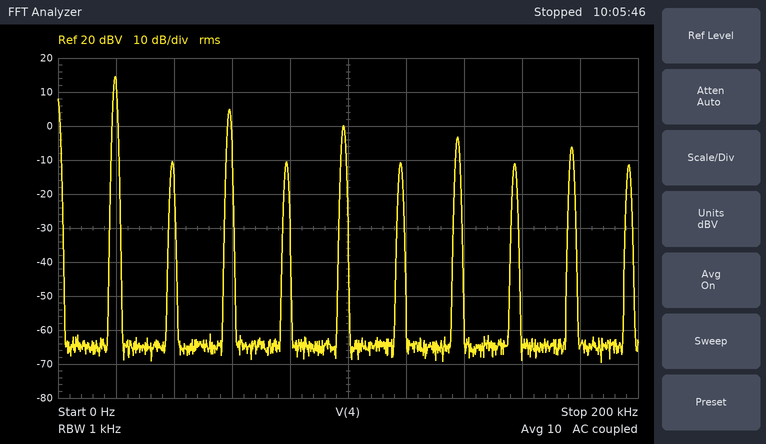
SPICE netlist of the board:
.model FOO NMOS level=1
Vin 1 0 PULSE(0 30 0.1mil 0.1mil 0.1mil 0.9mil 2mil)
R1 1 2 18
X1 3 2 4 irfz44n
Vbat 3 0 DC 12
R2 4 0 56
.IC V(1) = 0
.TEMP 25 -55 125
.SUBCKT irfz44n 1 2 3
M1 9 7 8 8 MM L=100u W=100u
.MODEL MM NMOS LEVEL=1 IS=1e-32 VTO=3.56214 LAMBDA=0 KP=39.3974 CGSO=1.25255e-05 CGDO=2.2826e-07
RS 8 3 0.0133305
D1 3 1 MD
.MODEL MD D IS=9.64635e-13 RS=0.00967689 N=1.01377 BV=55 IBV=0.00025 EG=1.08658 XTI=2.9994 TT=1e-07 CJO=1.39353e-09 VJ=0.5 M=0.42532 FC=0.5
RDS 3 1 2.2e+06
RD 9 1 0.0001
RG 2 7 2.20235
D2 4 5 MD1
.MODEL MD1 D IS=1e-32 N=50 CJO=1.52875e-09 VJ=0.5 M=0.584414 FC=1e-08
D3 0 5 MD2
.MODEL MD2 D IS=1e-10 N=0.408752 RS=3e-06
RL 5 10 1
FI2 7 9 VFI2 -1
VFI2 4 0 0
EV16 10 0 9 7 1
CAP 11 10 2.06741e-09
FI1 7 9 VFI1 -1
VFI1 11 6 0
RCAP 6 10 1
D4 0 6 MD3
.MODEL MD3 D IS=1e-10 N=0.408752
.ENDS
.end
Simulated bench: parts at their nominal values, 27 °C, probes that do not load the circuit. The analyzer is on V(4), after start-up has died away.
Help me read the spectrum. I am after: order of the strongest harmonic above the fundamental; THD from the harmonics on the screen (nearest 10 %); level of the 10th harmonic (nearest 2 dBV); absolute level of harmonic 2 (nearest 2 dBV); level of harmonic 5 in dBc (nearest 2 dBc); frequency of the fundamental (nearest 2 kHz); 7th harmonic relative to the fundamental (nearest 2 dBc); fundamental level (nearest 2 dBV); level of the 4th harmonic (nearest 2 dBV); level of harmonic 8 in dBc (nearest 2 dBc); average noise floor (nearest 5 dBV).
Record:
3
40 %
-12 dBV
-10 dBV
-14 dBc
20 kHz
-18 dBc
14 dBV
-10 dBV
-26 dBc
-65 dBV
